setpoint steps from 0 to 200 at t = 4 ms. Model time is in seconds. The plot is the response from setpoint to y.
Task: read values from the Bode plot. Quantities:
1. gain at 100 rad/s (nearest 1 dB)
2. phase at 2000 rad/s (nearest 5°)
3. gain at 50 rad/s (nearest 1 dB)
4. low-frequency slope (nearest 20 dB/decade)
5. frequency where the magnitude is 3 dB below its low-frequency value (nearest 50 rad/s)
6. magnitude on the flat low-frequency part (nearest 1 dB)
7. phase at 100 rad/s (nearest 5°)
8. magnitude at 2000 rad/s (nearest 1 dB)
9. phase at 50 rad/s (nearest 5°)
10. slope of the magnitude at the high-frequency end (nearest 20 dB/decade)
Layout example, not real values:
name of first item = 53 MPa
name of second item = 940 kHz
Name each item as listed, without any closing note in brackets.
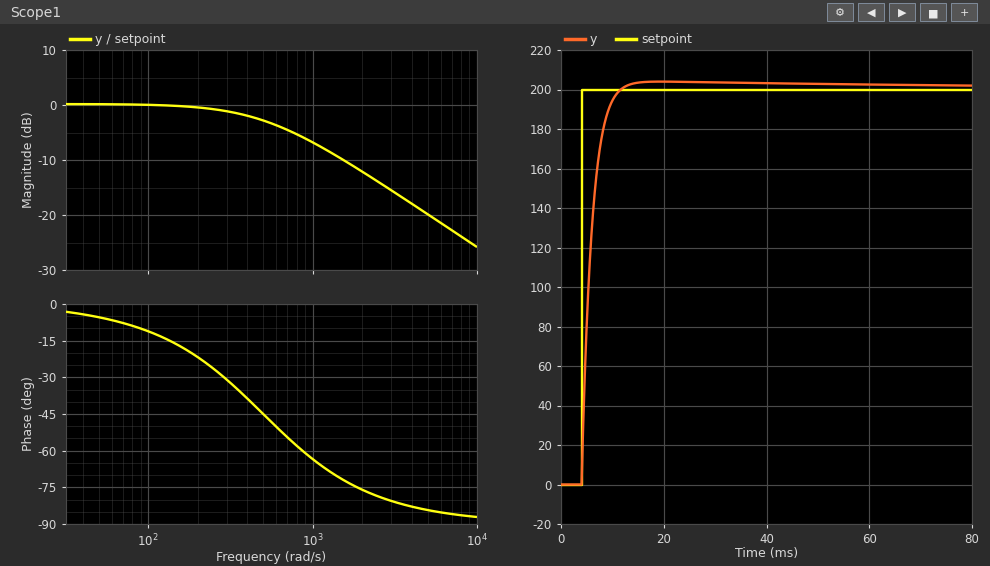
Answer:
gain at 100 rad/s = 0 dB
phase at 2000 rad/s = -75°
gain at 50 rad/s = 0 dB
low-frequency slope = 0 dB/decade
frequency where the magnitude is 3 dB below its low-frequency value = 500 rad/s
magnitude on the flat low-frequency part = 0 dB
phase at 100 rad/s = -10°
magnitude at 2000 rad/s = -12 dB
phase at 50 rad/s = -5°
slope of the magnitude at the high-frequency end = -20 dB/decade
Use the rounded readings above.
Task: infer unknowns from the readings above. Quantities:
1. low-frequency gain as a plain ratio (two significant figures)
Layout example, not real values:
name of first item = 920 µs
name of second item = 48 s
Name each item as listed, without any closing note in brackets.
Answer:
low-frequency gain as a plain ratio = 1.0
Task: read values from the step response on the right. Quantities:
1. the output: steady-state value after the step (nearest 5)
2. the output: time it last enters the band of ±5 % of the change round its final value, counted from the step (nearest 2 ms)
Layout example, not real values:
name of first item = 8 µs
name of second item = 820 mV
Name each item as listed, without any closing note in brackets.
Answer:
the output: steady-state value after the step = 200
the output: time it last enters the band of ±5 % of the change round its final value, counted from the step = 6 ms
